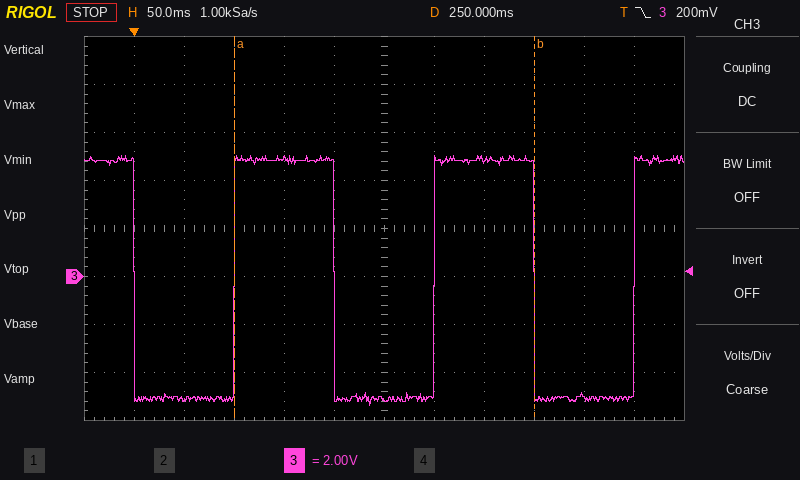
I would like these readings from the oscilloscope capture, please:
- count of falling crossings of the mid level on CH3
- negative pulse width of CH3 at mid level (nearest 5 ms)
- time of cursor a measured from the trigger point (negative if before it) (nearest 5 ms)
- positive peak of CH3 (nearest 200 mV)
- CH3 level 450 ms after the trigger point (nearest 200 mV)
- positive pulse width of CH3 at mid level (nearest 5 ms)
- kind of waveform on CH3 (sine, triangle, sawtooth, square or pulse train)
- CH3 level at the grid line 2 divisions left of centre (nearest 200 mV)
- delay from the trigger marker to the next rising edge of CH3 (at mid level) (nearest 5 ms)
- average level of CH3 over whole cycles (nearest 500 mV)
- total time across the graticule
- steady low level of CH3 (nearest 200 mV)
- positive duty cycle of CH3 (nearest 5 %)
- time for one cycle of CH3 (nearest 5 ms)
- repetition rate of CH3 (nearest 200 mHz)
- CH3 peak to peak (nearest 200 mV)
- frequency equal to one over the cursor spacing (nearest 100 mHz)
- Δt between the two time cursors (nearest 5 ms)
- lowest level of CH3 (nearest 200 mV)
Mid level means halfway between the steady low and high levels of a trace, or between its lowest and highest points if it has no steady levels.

3
100 ms
+100 ms
5.0 V
-5.0 V
100 ms
square
5.0 V
100 ms
0.0 V
600 ms
-5.0 V
50 %
200 ms
5.0 Hz
10.4 V
3.3 Hz
300 ms
-5.4 V
